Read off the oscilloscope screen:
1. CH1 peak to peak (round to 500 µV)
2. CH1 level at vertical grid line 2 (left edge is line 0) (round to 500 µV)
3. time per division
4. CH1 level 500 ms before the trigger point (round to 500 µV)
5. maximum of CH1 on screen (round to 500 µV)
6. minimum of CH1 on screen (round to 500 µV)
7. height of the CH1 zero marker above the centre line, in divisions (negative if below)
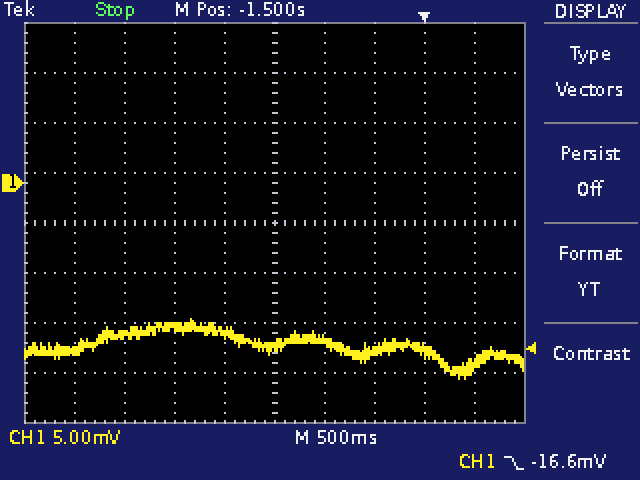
6.0 mV
-15.0 mV
500 ms
-17.0 mV
-13.5 mV
-19.5 mV
+0.8 div
